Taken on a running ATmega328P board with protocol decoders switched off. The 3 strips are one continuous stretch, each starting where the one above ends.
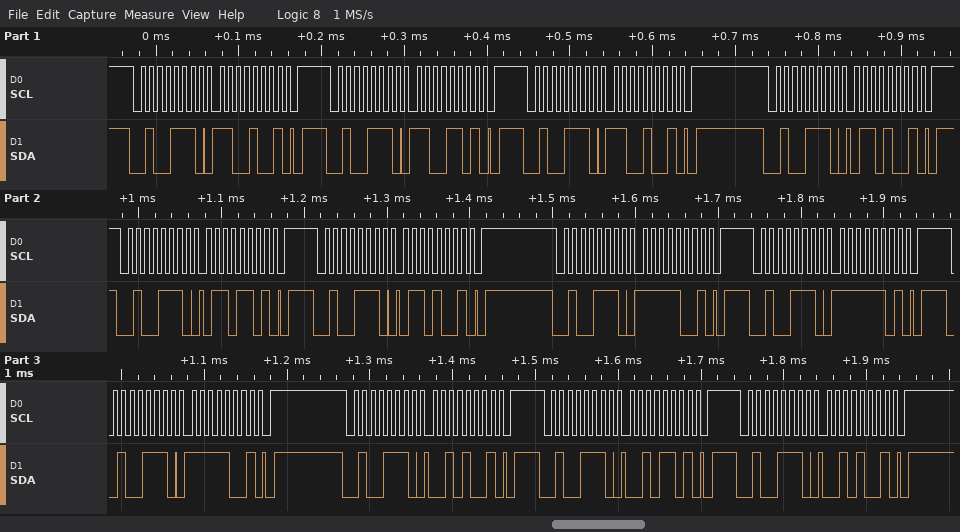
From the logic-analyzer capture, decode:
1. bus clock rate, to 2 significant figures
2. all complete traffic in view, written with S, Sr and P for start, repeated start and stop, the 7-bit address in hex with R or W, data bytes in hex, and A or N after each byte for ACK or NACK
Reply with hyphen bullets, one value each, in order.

- 100 kHz
- S 27W A C9 A P S 27W A CD A P S 27W A C9 A P S 27W A 69 A P S 27W A 6D A P S 27W A 69 A P S 27W A F9 A P S 27W A FD A P S 27W A F9 A P S 27W A 29 A P S 27W A 2D A P S 27W A 29 A P
